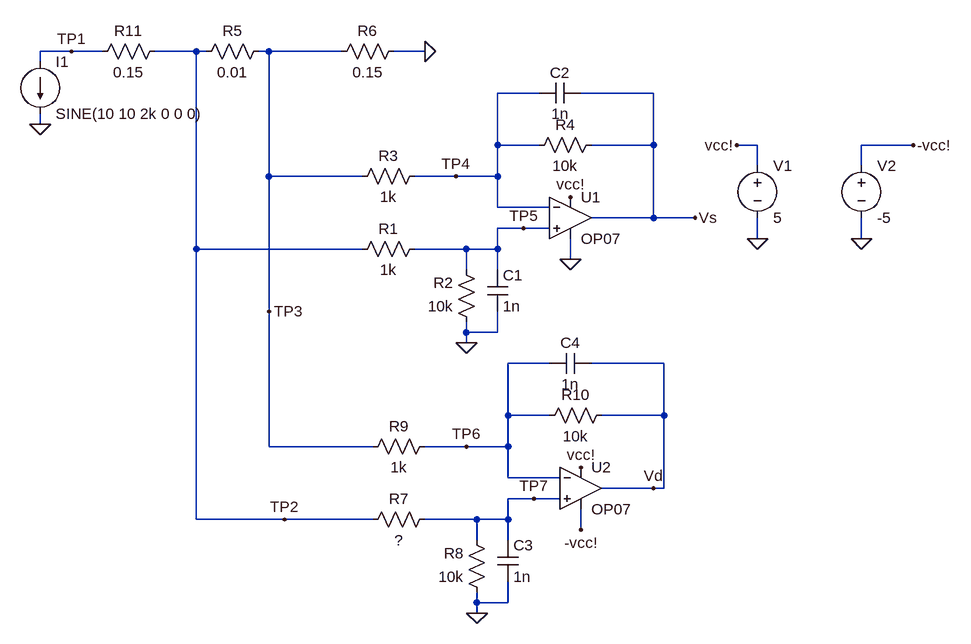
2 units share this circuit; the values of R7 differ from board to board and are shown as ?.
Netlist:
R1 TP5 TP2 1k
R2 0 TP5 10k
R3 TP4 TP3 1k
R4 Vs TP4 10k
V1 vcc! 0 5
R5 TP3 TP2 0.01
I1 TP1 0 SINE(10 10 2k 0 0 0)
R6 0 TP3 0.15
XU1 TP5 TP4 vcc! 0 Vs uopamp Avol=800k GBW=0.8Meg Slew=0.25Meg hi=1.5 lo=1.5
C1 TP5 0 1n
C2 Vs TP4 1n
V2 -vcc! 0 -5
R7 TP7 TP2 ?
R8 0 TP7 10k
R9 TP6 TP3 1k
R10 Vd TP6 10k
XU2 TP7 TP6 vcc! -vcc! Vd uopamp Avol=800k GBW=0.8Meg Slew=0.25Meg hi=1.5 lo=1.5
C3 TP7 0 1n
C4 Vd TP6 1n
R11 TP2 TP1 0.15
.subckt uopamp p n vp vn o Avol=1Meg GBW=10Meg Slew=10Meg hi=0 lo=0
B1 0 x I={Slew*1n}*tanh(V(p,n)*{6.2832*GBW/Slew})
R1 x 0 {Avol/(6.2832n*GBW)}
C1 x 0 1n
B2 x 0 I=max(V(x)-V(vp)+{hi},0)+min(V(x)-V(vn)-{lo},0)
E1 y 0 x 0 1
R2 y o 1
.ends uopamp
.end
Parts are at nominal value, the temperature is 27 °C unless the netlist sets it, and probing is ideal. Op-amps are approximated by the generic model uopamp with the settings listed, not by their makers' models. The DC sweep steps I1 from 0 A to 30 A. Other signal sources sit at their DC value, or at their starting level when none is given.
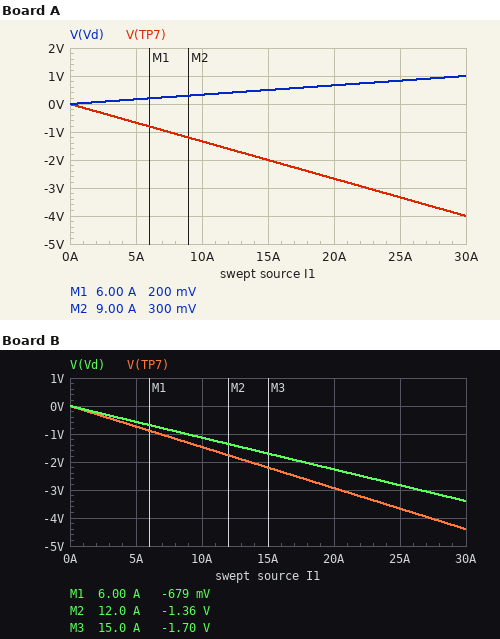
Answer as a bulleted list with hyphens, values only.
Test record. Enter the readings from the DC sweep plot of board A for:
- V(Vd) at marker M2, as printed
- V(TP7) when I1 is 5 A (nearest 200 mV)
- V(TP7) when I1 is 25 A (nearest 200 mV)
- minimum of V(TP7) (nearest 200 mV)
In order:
- 300 mV
- -600 mV
- -3.4 V
- -4.0 V
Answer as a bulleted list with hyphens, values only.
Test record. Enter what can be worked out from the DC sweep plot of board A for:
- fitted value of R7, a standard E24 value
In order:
- 2 kΩ
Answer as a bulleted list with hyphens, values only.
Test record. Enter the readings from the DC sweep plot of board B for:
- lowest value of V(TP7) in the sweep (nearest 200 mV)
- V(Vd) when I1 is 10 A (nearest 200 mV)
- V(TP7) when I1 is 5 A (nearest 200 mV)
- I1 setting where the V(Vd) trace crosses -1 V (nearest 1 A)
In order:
- -4.4 V
- -1.2 V
- -800 mV
- 9 A
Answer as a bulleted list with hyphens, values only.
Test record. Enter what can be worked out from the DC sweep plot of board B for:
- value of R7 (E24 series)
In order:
- 910 Ω
